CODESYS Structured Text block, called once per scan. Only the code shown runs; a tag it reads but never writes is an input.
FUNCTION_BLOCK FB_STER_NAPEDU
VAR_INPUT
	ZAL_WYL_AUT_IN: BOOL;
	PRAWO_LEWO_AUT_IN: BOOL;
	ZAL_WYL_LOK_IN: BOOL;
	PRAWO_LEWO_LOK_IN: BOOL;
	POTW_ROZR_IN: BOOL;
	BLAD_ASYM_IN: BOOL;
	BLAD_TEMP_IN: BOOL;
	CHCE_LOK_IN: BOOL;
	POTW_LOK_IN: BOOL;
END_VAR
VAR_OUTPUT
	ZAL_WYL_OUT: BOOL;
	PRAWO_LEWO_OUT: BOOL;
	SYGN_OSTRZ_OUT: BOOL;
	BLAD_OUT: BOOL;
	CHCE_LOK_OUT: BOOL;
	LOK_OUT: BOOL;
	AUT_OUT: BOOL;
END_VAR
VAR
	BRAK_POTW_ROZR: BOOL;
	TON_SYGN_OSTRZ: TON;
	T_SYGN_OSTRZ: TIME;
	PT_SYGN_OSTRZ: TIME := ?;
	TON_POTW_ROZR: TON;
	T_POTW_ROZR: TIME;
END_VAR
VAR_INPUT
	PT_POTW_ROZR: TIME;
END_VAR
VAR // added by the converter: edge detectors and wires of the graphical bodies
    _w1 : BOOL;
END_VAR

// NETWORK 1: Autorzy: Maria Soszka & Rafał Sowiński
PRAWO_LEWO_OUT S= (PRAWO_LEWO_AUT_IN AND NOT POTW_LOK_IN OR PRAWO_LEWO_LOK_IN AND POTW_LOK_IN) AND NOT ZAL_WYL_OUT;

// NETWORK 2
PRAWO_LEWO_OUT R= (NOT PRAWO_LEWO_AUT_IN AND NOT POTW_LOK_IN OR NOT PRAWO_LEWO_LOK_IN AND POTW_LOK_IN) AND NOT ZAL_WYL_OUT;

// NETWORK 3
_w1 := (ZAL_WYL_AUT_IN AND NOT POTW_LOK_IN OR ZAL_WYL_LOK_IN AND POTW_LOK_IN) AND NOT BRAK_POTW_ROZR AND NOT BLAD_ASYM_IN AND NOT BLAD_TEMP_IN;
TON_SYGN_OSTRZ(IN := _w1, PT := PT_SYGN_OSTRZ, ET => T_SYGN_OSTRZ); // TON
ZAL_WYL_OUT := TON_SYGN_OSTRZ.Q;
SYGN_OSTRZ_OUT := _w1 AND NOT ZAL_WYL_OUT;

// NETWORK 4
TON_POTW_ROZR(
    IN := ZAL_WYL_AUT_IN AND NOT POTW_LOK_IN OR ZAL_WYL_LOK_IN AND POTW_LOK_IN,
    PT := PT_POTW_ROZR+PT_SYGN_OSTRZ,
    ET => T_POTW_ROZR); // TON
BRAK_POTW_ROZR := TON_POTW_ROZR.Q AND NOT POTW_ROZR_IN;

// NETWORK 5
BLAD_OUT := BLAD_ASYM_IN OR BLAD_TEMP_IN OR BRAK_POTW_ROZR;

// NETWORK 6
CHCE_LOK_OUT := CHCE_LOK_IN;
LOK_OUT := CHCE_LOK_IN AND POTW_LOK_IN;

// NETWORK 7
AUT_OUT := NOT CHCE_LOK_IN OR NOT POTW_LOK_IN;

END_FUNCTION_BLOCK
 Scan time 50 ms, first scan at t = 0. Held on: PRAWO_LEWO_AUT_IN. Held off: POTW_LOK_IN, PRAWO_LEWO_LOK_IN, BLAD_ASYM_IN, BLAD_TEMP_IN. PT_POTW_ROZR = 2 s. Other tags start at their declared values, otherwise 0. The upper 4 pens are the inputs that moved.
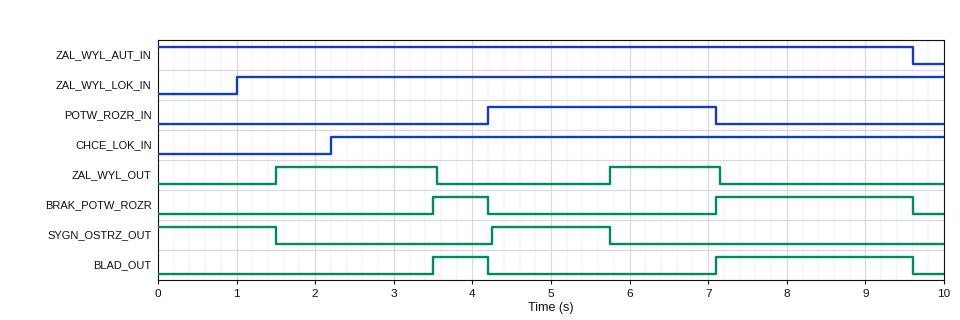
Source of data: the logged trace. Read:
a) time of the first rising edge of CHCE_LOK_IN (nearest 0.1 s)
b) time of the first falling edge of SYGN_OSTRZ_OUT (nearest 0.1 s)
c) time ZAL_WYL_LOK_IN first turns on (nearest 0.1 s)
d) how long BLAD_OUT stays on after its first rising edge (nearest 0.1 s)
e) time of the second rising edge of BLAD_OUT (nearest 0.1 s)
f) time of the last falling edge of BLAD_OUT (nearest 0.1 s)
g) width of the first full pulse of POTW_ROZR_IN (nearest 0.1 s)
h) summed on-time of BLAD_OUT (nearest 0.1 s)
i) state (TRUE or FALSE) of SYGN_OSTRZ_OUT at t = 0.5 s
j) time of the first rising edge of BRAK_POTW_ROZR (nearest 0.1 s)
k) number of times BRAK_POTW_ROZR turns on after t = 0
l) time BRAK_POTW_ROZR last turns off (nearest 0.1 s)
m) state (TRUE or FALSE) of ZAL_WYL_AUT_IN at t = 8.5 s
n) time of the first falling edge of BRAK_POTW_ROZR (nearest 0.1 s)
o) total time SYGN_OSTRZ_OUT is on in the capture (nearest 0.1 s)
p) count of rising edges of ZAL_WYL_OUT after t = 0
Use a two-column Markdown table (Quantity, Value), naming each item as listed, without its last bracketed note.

| Quantity | Value |
|---|---|
| time of the first rising edge of CHCE_LOK_IN | 2.2 s |
| time of the first falling edge of SYGN_OSTRZ_OUT | 1.5 s |
| time ZAL_WYL_LOK_IN first turns on | 1.0 s |
| how long BLAD_OUT stays on after its first rising edge | 0.7 s |
| time of the second rising edge of BLAD_OUT | 7.1 s |
| time of the last falling edge of BLAD_OUT | 9.6 s |
| width of the first full pulse of POTW_ROZR_IN | 2.9 s |
| summed on-time of BLAD_OUT | 3.2 s |
| state (TRUE or FALSE) of SYGN_OSTRZ_OUT at t = 0.5 s | TRUE |
| time of the first rising edge of BRAK_POTW_ROZR | 3.5 s |
| number of times BRAK_POTW_ROZR turns on after t = 0 | 2 |
| time BRAK_POTW_ROZR last turns off | 9.6 s |
| state (TRUE or FALSE) of ZAL_WYL_AUT_IN at t = 8.5 s | TRUE |
| time of the first falling edge of BRAK_POTW_ROZR | 4.2 s |
| total time SYGN_OSTRZ_OUT is on in the capture | 3.0 s |
| count of rising edges of ZAL_WYL_OUT after t = 0 | 2 |
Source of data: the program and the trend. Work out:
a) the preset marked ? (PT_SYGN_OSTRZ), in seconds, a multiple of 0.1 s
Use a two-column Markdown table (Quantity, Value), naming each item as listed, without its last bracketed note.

| Quantity | Value |
|---|---|
| the preset marked ? (PT_SYGN_OSTRZ), in seconds, a multiple of 0.1 s | 1.5 s |
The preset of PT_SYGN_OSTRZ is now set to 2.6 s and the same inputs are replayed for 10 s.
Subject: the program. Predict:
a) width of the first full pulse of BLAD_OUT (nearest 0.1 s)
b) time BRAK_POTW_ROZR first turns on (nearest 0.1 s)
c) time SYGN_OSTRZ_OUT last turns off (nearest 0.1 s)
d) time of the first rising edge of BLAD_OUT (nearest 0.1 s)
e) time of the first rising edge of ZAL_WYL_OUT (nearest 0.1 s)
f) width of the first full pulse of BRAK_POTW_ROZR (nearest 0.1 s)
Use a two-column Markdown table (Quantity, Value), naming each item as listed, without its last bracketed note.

| Quantity | Value |
|---|---|
| width of the first full pulse of BLAD_OUT | 2.5 s |
| time BRAK_POTW_ROZR first turns on | 7.1 s |
| time SYGN_OSTRZ_OUT last turns off | 2.6 s |
| time of the first rising edge of BLAD_OUT | 7.1 s |
| time of the first rising edge of ZAL_WYL_OUT | 2.6 s |
| width of the first full pulse of BRAK_POTW_ROZR | 2.5 s |
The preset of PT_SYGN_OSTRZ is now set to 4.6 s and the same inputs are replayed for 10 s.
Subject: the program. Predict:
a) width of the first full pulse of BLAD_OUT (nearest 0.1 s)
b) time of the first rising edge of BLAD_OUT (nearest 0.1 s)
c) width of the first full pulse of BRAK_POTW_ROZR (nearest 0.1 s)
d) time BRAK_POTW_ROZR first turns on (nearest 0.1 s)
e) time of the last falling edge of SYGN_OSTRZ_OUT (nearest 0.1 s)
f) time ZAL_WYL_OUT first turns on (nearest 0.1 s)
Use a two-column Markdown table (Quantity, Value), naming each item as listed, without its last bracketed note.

| Quantity | Value |
|---|---|
| width of the first full pulse of BLAD_OUT | 2.5 s |
| time of the first rising edge of BLAD_OUT | 7.1 s |
| width of the first full pulse of BRAK_POTW_ROZR | 2.5 s |
| time BRAK_POTW_ROZR first turns on | 7.1 s |
| time of the last falling edge of SYGN_OSTRZ_OUT | 4.6 s |
| time ZAL_WYL_OUT first turns on | 4.6 s |
